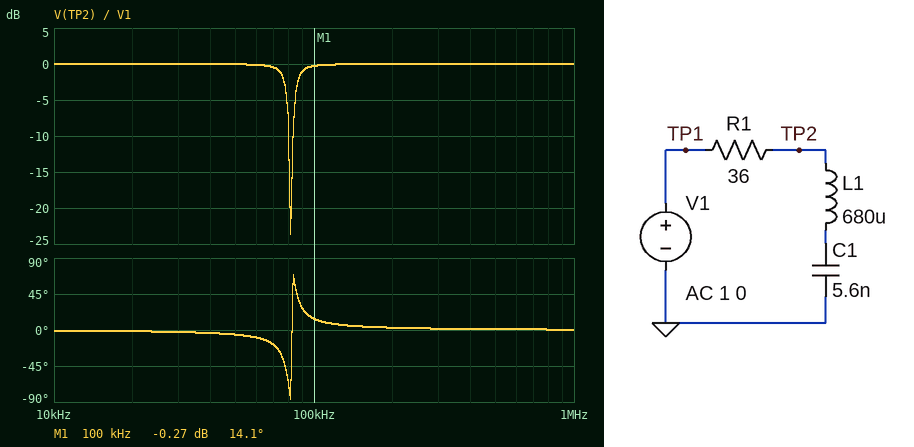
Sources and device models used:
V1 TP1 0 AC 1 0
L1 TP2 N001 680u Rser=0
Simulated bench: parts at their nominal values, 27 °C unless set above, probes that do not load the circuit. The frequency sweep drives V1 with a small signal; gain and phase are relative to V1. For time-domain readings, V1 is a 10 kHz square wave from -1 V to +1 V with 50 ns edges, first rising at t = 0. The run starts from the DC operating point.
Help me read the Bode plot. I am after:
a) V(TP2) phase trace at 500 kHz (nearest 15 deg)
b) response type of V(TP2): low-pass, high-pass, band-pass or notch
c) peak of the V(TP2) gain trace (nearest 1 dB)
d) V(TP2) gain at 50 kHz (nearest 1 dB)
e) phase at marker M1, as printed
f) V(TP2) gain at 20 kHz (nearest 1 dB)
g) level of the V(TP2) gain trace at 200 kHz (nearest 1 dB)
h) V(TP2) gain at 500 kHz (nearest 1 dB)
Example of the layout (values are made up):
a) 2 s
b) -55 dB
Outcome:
a) 0 deg
b) notch
c) 0 dB
d) 0 dB
e) 14.1 deg
f) 0 dB
g) 0 dB
h) 0 dB
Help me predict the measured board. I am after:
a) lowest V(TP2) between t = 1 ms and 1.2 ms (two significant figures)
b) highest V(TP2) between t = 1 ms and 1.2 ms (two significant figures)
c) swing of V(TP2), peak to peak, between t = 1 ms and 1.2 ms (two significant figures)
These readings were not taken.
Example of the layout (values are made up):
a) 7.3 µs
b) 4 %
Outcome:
a) -1.1 V
b) 1.1 V
c) 2.3 V
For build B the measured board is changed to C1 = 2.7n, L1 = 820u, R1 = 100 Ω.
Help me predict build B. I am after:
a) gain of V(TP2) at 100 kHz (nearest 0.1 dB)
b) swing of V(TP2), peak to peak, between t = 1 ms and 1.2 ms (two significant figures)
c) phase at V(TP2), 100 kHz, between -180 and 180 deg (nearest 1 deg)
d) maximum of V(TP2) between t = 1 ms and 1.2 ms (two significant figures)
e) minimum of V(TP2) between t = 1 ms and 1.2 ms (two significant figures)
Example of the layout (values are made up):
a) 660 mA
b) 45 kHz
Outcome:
a) -4.5 dB
b) 2.5 V
c) -53 deg
d) 1.2 V
e) -1.2 V
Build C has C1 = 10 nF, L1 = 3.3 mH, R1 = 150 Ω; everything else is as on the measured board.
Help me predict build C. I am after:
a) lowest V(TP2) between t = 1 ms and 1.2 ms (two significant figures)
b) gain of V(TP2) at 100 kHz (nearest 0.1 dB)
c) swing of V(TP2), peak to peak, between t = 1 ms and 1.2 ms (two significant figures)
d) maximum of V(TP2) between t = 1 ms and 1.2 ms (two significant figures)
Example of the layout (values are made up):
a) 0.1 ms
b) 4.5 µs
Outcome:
a) -1.3 V
b) 0 dB
c) 2.7 V
d) 1.3 V
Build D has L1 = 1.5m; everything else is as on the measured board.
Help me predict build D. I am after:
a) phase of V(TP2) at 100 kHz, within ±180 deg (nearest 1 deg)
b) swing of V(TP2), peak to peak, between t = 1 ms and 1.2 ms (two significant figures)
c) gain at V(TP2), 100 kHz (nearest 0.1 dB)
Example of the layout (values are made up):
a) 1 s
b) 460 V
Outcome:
a) 3 deg
b) 2.2 V
c) 0 dB
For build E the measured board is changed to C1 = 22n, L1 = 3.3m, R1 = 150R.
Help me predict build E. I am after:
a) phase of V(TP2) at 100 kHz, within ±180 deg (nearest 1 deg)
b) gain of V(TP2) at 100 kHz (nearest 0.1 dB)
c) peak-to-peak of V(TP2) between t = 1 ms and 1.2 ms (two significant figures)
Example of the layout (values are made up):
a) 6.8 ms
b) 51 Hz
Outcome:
a) 4 deg
b) 0 dB
c) 2.5 V
